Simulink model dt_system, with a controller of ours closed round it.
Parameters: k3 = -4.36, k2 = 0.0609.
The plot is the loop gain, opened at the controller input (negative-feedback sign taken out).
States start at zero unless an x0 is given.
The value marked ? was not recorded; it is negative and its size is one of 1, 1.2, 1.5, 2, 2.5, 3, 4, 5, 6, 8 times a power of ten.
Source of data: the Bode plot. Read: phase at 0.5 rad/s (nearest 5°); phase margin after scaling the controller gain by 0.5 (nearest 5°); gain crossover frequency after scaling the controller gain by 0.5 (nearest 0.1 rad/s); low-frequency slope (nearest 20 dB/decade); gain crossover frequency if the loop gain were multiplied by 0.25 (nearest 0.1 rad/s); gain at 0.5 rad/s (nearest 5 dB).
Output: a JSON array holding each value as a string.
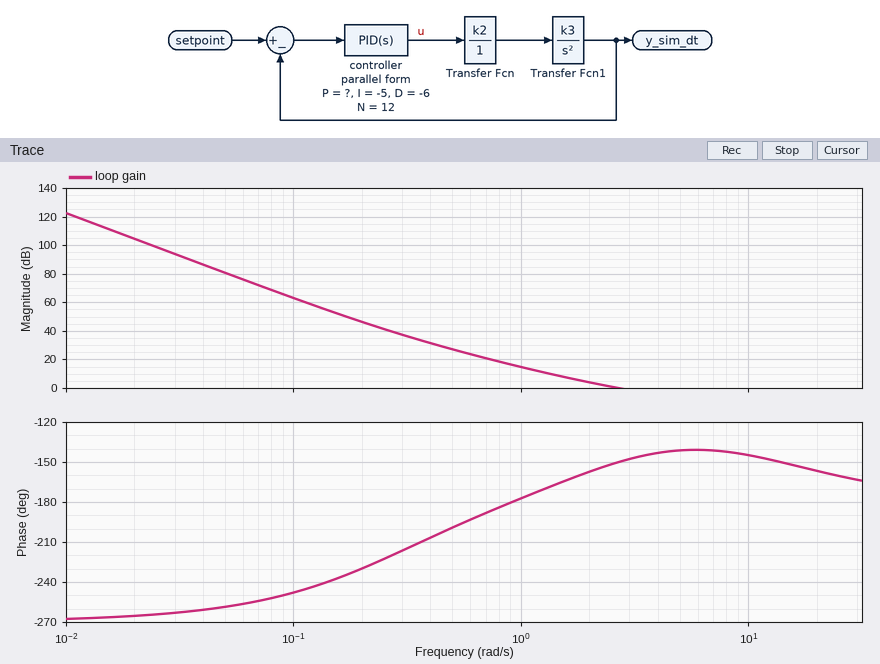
["-200°", "20°", "1.7 rad/s", "-60 dB/decade", "1.2 rad/s", "25 dB"]
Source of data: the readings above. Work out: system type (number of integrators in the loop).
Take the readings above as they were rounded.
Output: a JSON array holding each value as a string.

["3"]
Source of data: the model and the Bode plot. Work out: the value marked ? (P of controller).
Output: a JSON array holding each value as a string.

["-20"]
